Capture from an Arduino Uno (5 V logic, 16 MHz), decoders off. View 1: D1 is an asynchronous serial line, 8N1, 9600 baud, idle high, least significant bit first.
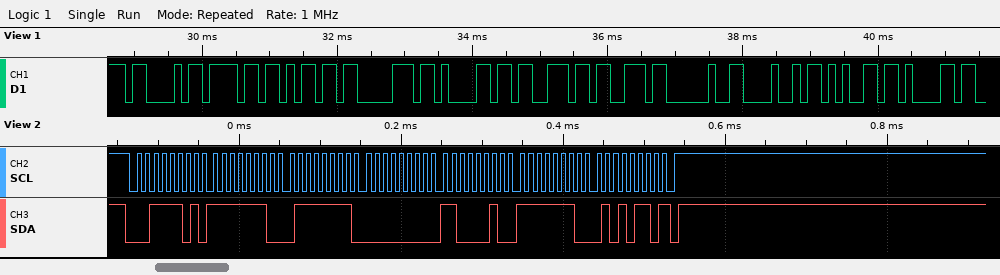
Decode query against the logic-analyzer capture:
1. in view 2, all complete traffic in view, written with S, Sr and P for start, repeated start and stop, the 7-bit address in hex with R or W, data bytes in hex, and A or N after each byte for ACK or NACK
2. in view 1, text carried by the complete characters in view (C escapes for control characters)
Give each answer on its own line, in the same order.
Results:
S 1ER A FE A 7F A 00 A C2 A FE A 56 N P
"Compass Hea"
